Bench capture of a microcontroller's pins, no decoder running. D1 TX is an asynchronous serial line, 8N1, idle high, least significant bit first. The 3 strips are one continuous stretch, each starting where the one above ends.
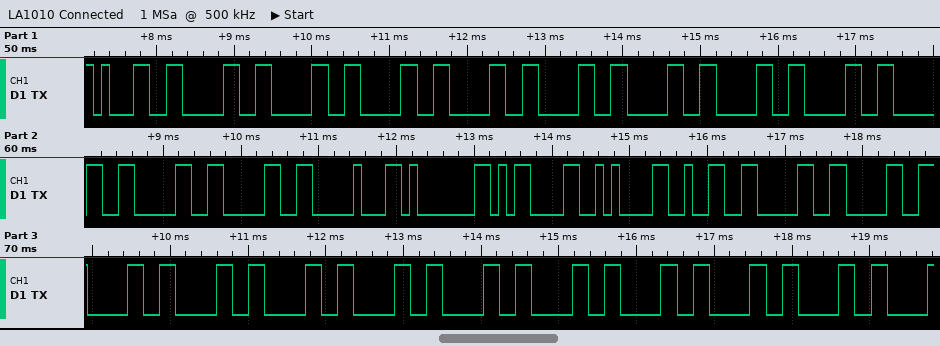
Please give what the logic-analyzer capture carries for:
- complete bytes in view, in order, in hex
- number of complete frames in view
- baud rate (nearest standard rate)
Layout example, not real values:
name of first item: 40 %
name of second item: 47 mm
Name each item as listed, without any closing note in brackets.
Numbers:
complete bytes in view, in order, in hex: 31 30 30 30 30 30 30 30 30 30 30 30 10 01 0D 0A 32 30 30 30 30 30 30 30 30 30 30 30
number of complete frames in view: 28
baud rate: 9600 baud
